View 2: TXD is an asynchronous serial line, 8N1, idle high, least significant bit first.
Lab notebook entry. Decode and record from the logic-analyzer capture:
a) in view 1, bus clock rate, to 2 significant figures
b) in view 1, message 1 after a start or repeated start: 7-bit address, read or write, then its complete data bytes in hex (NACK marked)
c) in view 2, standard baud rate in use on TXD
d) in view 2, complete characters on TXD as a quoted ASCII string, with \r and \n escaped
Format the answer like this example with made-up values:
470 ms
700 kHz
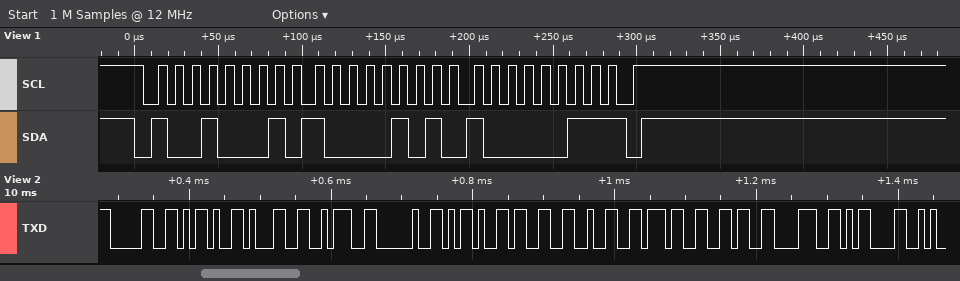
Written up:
100 kHz
0x48 read: 85 83 NACK
115200 baud
"0-1: -32768\r"
